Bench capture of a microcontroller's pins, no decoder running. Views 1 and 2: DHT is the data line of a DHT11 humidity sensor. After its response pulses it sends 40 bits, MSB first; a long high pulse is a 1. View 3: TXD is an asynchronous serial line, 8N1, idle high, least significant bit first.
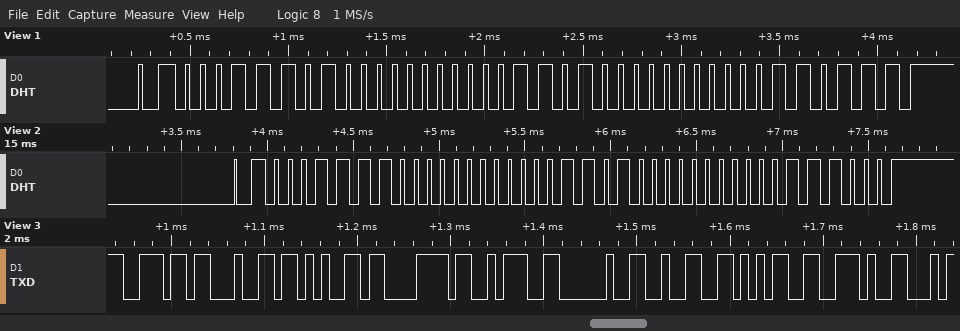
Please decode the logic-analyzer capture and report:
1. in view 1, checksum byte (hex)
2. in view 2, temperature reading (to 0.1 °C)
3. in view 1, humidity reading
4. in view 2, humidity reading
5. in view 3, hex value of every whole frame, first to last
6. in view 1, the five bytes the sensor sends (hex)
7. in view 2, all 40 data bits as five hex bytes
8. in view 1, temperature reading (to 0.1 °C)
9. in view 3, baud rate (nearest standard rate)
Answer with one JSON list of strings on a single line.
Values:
["0x37", "26.0 °C", "29 %", "30 %", "6E 64 65 78 3A 20 32 35 2E", "1D 00 1A 00 37", "1E 00 1A 00 38", "26.0 °C", "115200 baud"]
